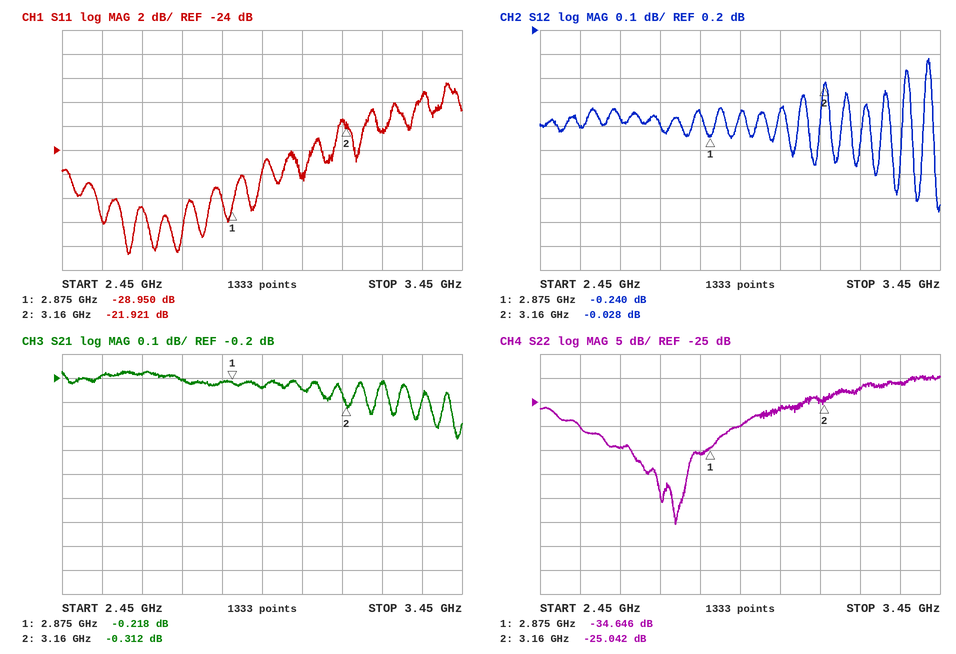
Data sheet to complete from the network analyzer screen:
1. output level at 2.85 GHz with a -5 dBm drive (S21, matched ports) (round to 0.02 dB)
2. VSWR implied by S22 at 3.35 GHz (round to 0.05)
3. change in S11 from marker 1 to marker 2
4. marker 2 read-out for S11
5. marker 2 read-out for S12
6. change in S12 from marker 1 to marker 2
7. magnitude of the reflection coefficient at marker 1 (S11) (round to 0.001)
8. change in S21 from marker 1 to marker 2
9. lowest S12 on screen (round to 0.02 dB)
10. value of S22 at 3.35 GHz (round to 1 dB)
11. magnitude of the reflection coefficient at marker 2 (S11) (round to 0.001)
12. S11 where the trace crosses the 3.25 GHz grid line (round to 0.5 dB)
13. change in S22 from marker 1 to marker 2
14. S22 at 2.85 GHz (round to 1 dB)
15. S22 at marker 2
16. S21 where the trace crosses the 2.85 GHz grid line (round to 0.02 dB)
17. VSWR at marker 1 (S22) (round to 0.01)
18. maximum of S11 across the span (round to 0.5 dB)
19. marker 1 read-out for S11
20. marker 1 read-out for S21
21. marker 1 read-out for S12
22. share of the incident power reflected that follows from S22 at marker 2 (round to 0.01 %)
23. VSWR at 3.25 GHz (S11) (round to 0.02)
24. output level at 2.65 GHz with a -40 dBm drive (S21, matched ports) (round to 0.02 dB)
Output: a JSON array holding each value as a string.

["-5.22 dBm", "1.20", "7.029 dB", "-21.921 dB", "-0.028 dB", "0.212 dB", "0.036", "-0.094 dB", "-0.56 dB", "-21 dB", "0.080", "-22.5 dB", "9.604 dB", "-36 dB", "-25.042 dB", "-0.22 dB", "1.04", "-18.5 dB", "-28.950 dB", "-0.218 dB", "-0.240 dB", "0.31 %", "1.16", "-40.18 dBm"]
